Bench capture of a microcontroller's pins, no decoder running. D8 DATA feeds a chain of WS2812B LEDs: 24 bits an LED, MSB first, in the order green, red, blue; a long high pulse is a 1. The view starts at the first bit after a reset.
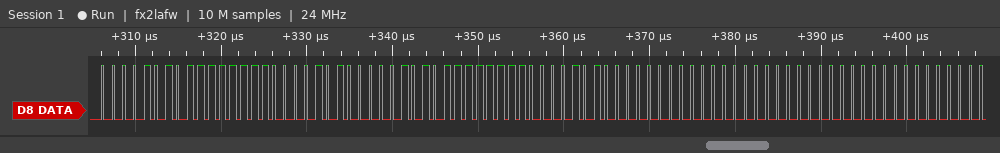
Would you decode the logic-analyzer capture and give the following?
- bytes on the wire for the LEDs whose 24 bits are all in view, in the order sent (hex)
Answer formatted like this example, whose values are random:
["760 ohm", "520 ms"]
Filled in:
["0A FF 0A 0A FF 0A 00 00 00"]
